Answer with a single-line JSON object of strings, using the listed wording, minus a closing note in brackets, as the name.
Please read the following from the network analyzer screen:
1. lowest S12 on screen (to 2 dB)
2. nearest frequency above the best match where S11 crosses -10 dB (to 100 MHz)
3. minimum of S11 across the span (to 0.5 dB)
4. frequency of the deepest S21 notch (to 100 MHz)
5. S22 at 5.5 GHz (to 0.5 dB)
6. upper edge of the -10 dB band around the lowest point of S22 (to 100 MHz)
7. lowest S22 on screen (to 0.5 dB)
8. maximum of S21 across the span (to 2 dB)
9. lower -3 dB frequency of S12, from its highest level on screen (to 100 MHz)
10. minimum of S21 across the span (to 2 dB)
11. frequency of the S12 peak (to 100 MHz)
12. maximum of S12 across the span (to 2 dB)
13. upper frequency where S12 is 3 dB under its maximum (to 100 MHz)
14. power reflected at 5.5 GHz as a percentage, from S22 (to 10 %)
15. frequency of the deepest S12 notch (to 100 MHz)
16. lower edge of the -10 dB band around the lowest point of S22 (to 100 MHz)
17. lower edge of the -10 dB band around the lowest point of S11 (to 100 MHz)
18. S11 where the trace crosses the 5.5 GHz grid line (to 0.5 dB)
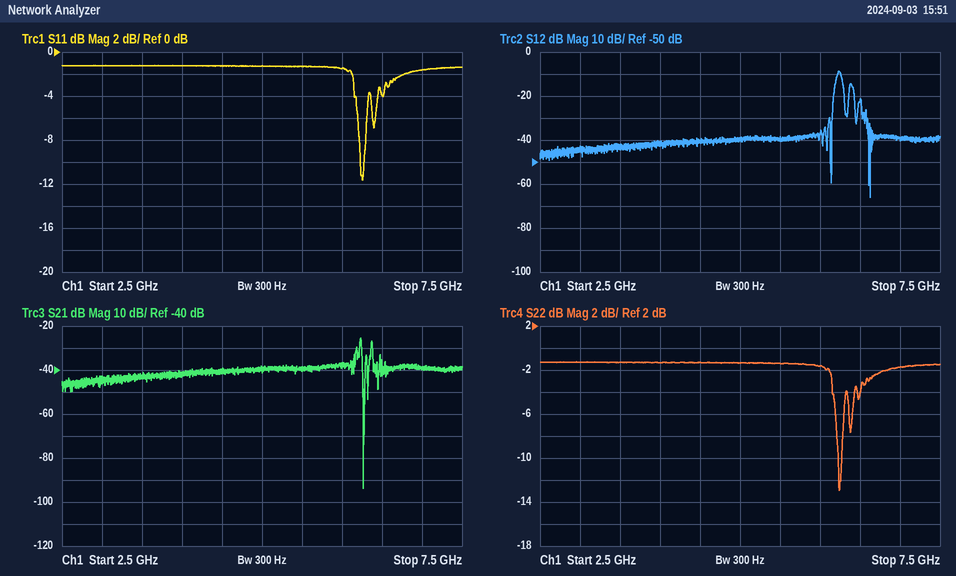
{"lowest S12 on screen": "-66 dB", "nearest frequency above the best match where S11 crosses -10 dB": "6.3 GHz", "minimum of S11 across the span": "-11.5 dB", "frequency of the deepest S21 notch": "6.3 GHz", "S22 at 5.5 GHz": "-1.5 dB", "upper edge of the -10 dB band around the lowest point of S22": "6.3 GHz", "lowest S22 on screen": "-13.0 dB", "maximum of S21 across the span": "-26 dB", "lower -3 dB frequency of S12, from its highest level on screen": "6.2 GHz", "minimum of S21 across the span": "-94 dB", "frequency of the S12 peak": "6.2 GHz", "maximum of S12 across the span": "-8 dB", "upper frequency where S12 is 3 dB under its maximum": "6.3 GHz", "power reflected at 5.5 GHz as a percentage, from S22": "70 %", "frequency of the deepest S12 notch": "6.6 GHz", "lower edge of the -10 dB band around the lowest point of S22": "6.2 GHz", "lower edge of the -10 dB band around the lowest point of S11": "6.2 GHz", "S11 where the trace crosses the 5.5 GHz grid line": "-1.5 dB"}
